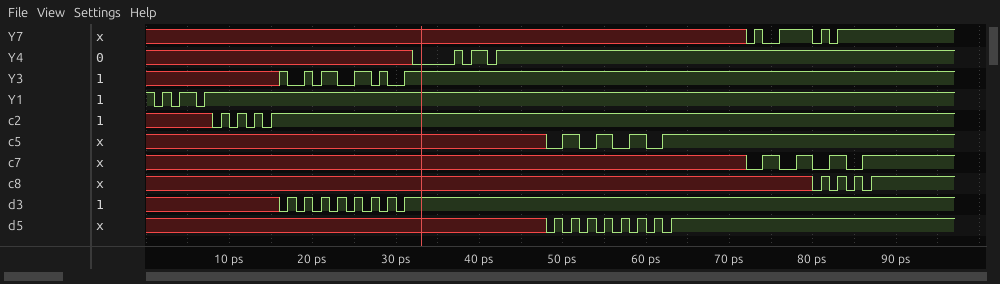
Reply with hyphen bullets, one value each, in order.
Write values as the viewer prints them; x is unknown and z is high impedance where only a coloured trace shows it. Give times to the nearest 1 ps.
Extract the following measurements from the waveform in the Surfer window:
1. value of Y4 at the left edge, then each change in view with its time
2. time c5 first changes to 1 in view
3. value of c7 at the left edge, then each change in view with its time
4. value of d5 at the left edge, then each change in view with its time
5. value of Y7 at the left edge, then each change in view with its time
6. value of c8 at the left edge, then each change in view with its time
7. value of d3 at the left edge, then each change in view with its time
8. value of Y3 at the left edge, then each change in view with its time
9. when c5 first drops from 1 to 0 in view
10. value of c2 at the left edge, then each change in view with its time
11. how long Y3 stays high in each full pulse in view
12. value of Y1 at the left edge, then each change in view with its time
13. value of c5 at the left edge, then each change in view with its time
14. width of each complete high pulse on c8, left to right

- x, 0 at 32 ps, 1 at 37 ps, 0 at 38 ps, 1 at 39 ps, 0 at 41 ps, 1 at 42 ps
- 50 ps
- x, 0 at 72 ps, 1 at 74 ps, 0 at 76 ps, 1 at 78 ps, 0 at 80 ps, 1 at 82 ps, 0 at 84 ps, 1 at 86 ps
- x, 0 at 48 ps, 1 at 49 ps, 0 at 50 ps, 1 at 51 ps, 0 at 52 ps, 1 at 53 ps, 0 at 54 ps, 1 at 55 ps, 0 at 56 ps, 1 at 57 ps, 0 at 58 ps, 1 at 59 ps, 0 at 60 ps, 1 at 61 ps, 0 at 62 ps, 1 at 63 ps
- x, 0 at 72 ps, 1 at 73 ps, 0 at 74 ps, 1 at 76 ps, 0 at 80 ps, 1 at 81 ps, 0 at 82 ps, 1 at 83 ps
- x, 0 at 80 ps, 1 at 81 ps, 0 at 82 ps, 1 at 83 ps, 0 at 84 ps, 1 at 85 ps, 0 at 86 ps, 1 at 87 ps
- x, 0 at 16 ps, 1 at 17 ps, 0 at 18 ps, 1 at 19 ps, 0 at 20 ps, 1 at 21 ps, 0 at 22 ps, 1 at 23 ps, 0 at 24 ps, 1 at 25 ps, 0 at 26 ps, 1 at 27 ps, 0 at 28 ps, 1 at 29 ps, 0 at 30 ps, 1 at 31 ps
- x, 1 at 16 ps, 0 at 17 ps, 1 at 19 ps, 0 at 20 ps, 1 at 21 ps, 0 at 23 ps, 1 at 25 ps, 0 at 27 ps, 1 at 28 ps, 0 at 29 ps, 1 at 31 ps
- 52 ps
- x, 0 at 8 ps, 1 at 9 ps, 0 at 10 ps, 1 at 11 ps, 0 at 12 ps, 1 at 13 ps, 0 at 14 ps, 1 at 15 ps
- 1 ps, 2 ps, 2 ps, 1 ps
- 1, 0 at 1 ps, 1 at 2 ps, 0 at 3 ps, 1 at 4 ps, 0 at 6 ps, 1 at 7 ps
- x, 0 at 48 ps, 1 at 50 ps, 0 at 52 ps, 1 at 54 ps, 0 at 56 ps, 1 at 58 ps, 0 at 60 ps, 1 at 62 ps
- 1 ps, 1 ps, 1 ps
